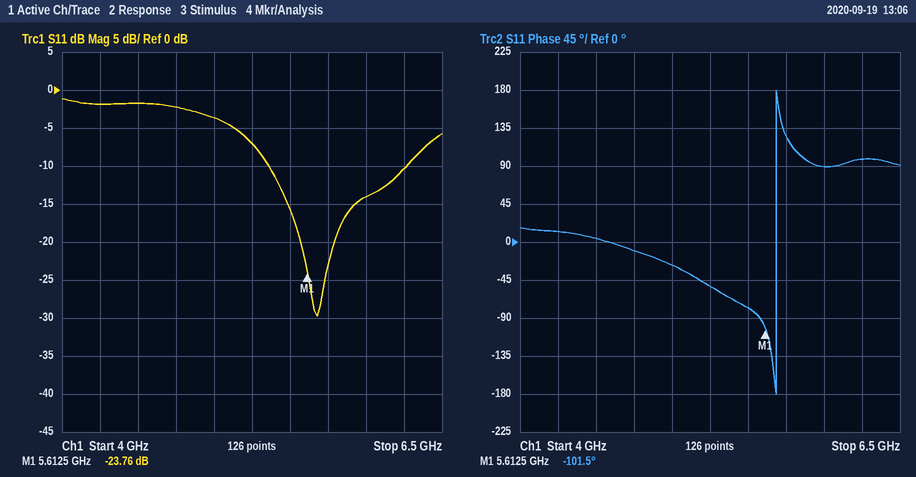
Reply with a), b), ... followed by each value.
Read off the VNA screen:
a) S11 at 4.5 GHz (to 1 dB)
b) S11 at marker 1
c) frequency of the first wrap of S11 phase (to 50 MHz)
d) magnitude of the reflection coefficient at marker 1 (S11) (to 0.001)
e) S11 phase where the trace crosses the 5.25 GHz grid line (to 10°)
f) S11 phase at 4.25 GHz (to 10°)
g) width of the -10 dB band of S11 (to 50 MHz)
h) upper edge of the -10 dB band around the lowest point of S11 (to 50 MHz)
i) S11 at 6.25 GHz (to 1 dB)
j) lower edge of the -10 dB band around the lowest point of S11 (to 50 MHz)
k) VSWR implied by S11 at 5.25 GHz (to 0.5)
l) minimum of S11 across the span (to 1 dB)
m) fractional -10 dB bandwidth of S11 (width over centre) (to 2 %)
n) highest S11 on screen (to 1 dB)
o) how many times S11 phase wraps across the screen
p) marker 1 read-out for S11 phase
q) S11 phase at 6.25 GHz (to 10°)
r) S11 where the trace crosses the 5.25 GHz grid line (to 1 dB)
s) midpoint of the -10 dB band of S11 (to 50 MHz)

a) -2 dB
b) -23.76 dB
c) 5.70 GHz
d) 0.065
e) -50°
f) 10°
g) 900 MHz
h) 6.25 GHz
i) -10 dB
j) 5.35 GHz
k) 2.5
l) -30 dB
m) 16 %
n) -1 dB
o) 1
p) -101.5°
q) 100°
r) -7 dB
s) 5.80 GHz
